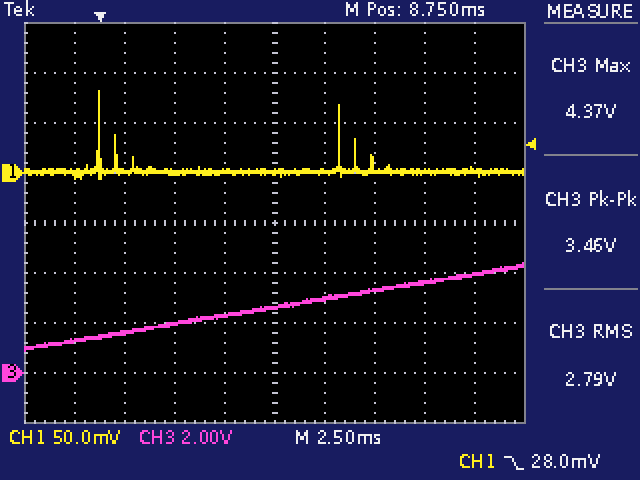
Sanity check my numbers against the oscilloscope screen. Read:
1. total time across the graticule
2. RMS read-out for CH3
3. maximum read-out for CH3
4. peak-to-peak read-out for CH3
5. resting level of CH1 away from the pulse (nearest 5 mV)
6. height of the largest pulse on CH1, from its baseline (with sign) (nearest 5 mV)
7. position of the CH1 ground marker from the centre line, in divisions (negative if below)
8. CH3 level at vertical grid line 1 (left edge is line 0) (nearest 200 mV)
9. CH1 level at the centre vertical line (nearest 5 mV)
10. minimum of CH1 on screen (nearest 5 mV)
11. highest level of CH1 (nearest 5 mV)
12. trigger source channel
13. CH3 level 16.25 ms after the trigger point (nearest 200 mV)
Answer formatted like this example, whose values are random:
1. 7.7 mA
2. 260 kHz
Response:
1. 25 ms
2. 2.79 V
3. 4.37 V
4. 3.46 V
5. 0 mV
6. +80 mV
7. +1.0 div
8. 1.2 V
9. 0 mV
10. -5 mV
11. 80 mV
12. CH1
13. 3.6 V
